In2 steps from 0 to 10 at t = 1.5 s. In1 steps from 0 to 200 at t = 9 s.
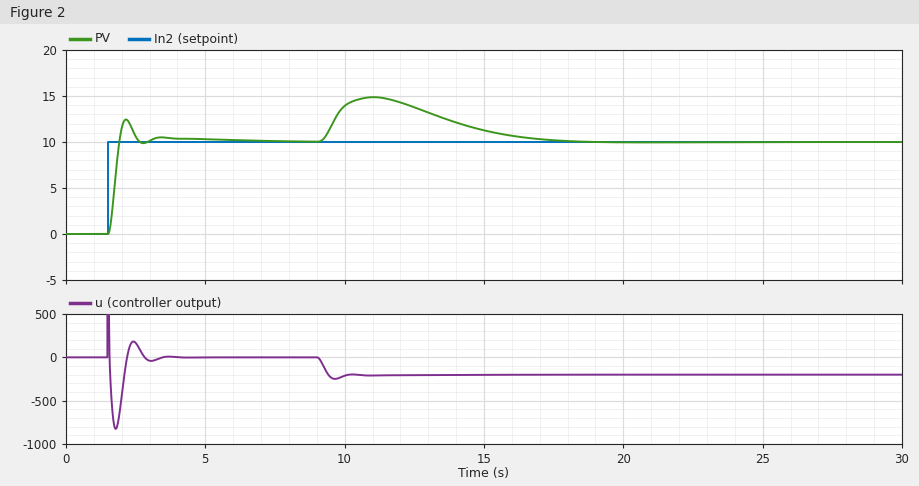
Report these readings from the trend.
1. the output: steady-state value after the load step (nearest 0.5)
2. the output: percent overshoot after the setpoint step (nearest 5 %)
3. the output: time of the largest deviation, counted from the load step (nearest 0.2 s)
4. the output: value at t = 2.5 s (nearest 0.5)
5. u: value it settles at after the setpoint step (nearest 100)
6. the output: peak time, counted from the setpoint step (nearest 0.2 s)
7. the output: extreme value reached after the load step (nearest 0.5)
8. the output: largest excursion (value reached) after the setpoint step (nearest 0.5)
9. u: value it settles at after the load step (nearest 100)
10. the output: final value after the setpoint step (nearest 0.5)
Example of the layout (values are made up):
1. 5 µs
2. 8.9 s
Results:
1. 10.0
2. 25 %
3. 2.0 s
4. 10.5
5. 0
6. 0.6 s
7. 15.0
8. 12.5
9. -200
10. 10.0
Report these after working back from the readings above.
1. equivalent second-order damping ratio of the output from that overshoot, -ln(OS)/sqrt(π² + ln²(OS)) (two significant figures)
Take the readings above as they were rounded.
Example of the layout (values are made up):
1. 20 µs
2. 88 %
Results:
1. 0.40
